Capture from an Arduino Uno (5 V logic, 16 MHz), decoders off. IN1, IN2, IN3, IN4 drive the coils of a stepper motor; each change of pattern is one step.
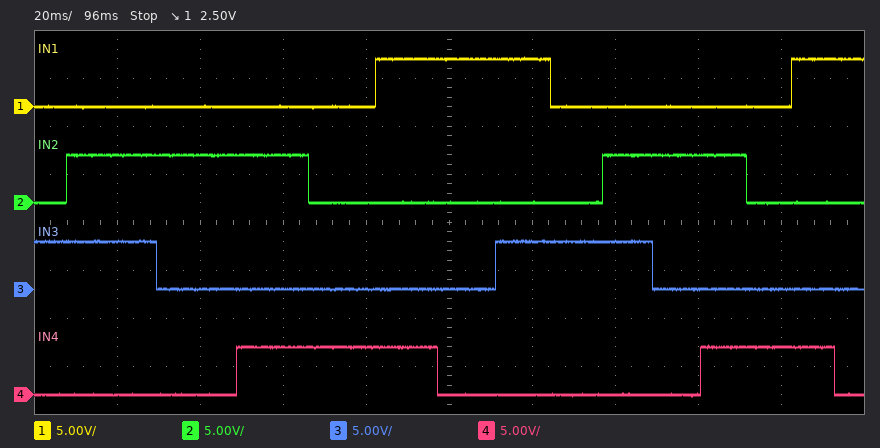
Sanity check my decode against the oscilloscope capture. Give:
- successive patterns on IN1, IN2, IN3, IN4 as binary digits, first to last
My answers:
0010 0110 0100 0101 0001 1001 1000 1010 0010 0110 0100 0101 0001 1001 1000
